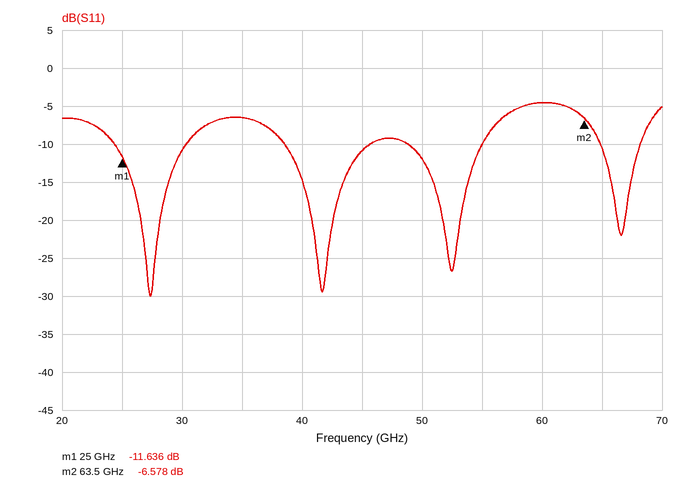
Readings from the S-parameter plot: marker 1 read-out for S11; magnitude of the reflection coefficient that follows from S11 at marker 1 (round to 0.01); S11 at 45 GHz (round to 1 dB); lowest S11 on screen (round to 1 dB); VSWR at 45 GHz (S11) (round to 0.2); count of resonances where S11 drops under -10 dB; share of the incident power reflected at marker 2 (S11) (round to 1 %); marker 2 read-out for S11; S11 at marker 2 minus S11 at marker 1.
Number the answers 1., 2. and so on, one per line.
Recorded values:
1. -11.636 dB
2. 0.26
3. -11 dB
4. -30 dB
5. 1.8
6. 4
7. 22 %
8. -6.578 dB
9. 5.058 dB
